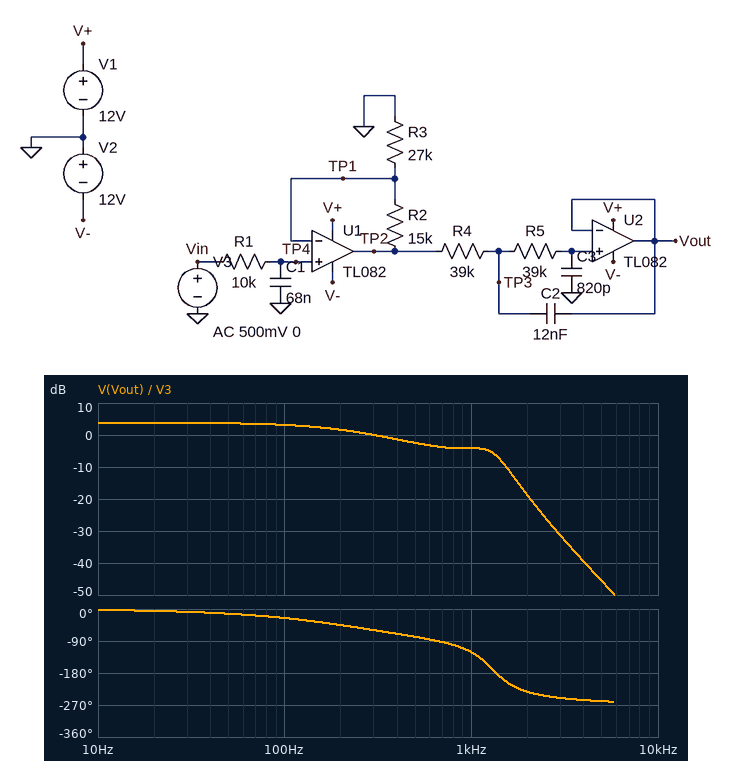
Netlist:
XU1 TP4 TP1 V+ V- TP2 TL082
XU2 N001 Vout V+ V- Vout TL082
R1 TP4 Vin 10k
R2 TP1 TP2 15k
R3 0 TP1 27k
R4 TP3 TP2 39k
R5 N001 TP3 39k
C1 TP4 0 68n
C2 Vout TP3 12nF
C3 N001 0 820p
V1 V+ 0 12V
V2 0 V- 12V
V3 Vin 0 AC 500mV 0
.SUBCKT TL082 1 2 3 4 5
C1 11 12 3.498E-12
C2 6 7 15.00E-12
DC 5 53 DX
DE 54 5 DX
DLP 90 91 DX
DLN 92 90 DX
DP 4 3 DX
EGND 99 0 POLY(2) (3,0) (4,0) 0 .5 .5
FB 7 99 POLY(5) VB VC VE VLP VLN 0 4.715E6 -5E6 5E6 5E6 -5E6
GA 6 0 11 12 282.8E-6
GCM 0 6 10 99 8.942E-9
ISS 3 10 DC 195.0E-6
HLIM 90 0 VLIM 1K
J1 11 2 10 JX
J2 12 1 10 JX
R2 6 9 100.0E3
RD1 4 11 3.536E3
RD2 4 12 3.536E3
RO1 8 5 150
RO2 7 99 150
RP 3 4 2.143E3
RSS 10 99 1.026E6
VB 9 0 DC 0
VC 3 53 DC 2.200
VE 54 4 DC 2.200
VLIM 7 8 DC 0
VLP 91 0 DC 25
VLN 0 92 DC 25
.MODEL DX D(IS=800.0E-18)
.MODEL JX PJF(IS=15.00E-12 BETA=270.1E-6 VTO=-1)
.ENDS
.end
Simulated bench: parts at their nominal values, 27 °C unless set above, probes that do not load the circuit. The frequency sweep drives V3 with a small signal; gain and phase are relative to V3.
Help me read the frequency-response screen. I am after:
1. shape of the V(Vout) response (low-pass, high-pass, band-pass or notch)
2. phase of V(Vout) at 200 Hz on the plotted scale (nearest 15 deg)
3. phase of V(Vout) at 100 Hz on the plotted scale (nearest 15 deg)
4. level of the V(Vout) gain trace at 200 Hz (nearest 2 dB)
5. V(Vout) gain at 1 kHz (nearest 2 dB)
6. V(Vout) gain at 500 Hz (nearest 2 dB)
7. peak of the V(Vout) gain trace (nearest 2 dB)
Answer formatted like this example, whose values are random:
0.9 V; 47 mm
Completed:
low-pass; -45 deg; -30 deg; 2 dB; -4 dB; -2 dB; 4 dB
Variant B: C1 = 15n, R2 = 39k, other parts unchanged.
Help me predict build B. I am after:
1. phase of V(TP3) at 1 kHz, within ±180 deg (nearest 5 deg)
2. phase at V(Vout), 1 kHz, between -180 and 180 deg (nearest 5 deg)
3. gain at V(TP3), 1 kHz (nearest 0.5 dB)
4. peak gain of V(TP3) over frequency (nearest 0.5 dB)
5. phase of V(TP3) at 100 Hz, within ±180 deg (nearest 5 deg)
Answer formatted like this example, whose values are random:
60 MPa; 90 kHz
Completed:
-75 deg; -90 deg; 10.0 dB; 10.5 dB; -5 deg
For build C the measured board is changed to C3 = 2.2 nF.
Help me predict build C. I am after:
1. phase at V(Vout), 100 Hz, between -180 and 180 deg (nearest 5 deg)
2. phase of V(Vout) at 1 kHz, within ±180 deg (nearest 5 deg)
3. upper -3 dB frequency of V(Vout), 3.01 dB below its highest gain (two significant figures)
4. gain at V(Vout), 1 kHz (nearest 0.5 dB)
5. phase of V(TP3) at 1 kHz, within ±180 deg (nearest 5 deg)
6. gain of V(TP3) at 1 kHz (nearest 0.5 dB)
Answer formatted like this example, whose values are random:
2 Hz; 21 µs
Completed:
-30 deg; 165 deg; 270 Hz; -11.0 dB; -165 deg; -9.5 dB
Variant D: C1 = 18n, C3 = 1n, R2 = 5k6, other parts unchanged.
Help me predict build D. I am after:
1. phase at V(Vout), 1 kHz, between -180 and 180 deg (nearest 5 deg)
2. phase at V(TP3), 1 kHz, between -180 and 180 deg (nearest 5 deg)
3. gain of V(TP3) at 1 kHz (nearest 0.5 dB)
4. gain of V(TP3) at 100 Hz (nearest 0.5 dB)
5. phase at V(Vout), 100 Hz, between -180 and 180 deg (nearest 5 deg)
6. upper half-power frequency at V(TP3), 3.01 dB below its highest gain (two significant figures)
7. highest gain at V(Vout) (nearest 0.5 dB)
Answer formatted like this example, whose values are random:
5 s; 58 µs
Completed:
-110 deg; -95 deg; 3.5 dB; 1.5 dB; -10 deg; 1.3 kHz; 3.0 dB
